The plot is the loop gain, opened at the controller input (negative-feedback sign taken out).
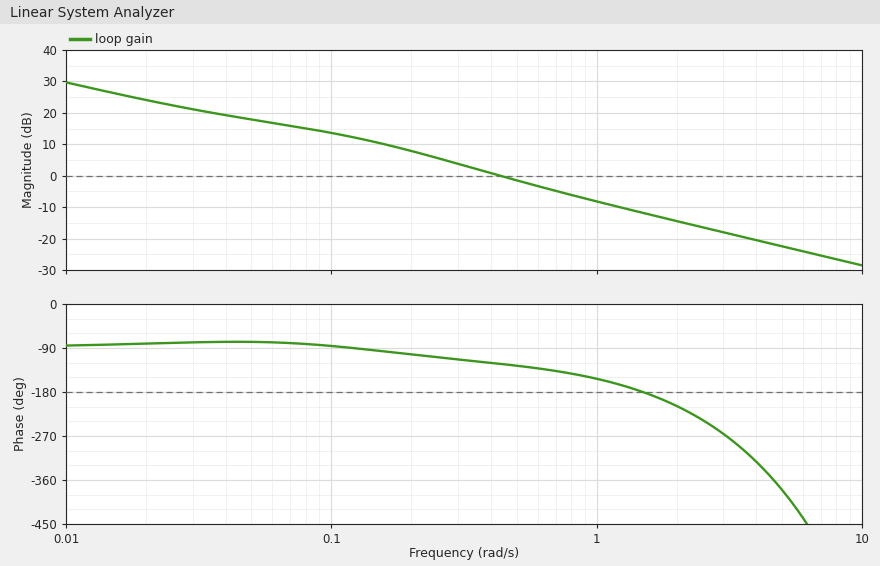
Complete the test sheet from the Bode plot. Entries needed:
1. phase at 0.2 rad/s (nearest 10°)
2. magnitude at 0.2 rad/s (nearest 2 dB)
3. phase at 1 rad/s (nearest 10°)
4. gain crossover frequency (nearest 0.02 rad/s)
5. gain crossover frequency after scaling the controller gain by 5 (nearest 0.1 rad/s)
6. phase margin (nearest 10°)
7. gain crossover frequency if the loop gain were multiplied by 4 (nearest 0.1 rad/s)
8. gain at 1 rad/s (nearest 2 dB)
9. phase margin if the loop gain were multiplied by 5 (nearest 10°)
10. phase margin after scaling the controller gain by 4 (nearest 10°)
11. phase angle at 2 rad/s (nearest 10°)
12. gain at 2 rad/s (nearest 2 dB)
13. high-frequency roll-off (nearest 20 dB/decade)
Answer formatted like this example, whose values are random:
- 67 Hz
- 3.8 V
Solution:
- -100°
- 8 dB
- -150°
- 0.44 rad/s
- 1.9 rad/s
- 60°
- 1.5 rad/s
- -8 dB
- -20°
- 0°
- -210°
- -14 dB
- -20 dB/decade
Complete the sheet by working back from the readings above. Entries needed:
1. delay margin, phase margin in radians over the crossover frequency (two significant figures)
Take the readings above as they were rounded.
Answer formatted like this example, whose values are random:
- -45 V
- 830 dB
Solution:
- 2.4 s
